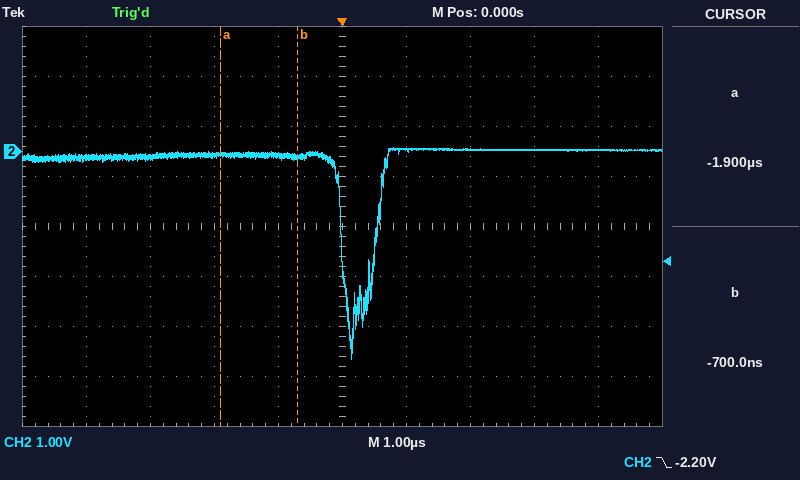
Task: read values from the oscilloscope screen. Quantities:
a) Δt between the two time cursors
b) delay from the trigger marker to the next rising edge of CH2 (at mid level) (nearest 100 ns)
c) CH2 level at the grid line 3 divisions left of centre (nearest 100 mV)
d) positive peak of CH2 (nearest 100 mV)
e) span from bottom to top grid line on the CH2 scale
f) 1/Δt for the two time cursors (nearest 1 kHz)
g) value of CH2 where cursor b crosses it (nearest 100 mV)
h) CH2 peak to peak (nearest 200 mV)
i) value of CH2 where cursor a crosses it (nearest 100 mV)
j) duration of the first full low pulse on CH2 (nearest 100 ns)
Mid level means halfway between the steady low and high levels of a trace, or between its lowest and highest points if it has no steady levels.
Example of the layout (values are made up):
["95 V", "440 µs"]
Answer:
["1.2 µs", "500 ns", "-100 mV", "100 mV", "8 V", "833 kHz", "-100 mV", "4.2 V", "-100 mV", "500 ns"]
